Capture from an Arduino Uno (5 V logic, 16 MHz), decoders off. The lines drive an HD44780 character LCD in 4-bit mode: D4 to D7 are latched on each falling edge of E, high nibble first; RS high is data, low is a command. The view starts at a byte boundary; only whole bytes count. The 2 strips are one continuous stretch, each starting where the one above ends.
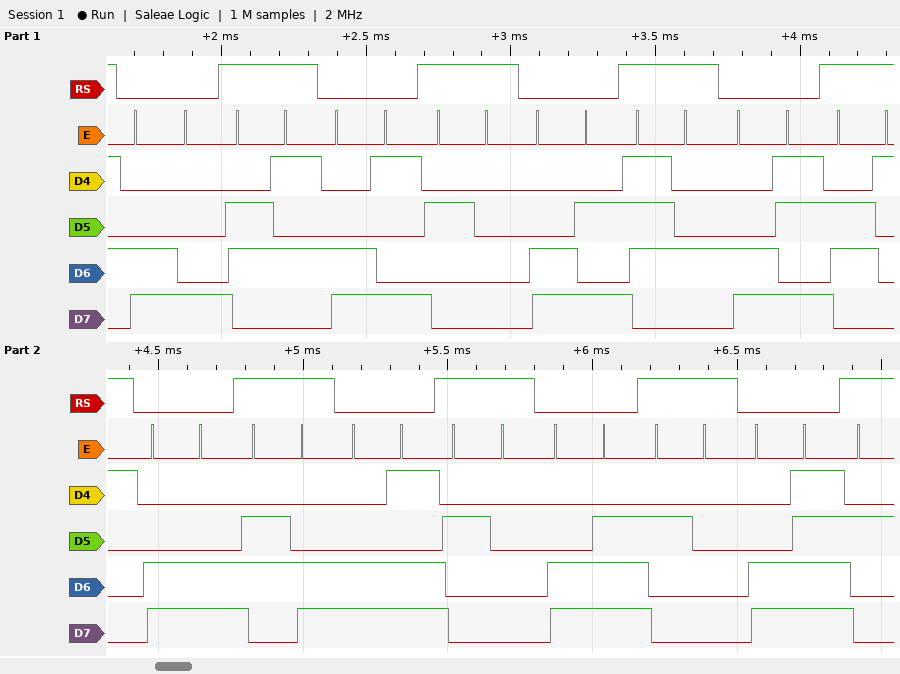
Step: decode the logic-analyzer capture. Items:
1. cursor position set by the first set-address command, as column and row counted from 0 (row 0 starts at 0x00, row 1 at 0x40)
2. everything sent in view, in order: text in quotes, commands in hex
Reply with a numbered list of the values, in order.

1. column 8, row 1
2. 0xC8 "e" 0xC9 " " 0xCA "t" 0xCB "a" 0xCC "l" 0xCD " " 0xCE " " 0xCF
